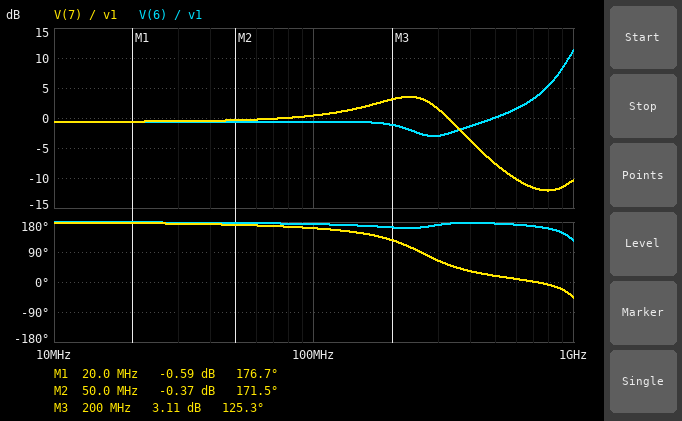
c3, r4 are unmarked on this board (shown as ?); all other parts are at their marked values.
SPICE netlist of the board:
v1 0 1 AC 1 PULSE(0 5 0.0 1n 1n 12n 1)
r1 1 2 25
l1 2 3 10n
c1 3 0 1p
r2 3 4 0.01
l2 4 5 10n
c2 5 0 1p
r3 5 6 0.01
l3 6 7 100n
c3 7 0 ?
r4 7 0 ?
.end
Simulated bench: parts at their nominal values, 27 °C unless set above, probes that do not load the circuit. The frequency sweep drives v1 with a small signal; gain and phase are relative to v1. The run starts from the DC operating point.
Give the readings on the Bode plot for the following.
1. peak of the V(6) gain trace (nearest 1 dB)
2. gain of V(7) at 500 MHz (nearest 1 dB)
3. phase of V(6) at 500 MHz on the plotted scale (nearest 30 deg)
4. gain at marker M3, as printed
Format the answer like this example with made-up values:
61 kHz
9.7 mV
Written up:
11 dB
-8 dB
180 deg
3.11 dB
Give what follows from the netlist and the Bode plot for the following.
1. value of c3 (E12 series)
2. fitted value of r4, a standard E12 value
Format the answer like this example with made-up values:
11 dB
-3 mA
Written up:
3.3 pF
330 Ω
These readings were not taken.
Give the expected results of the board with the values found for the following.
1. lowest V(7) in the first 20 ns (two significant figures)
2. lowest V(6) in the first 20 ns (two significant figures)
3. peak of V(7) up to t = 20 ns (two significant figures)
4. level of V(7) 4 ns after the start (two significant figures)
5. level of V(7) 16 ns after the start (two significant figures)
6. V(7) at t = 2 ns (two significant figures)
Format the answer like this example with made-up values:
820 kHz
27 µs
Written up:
-6.0 V
-5.0 V
1.4 V
-4.5 V
1.1 V
-5.3 V
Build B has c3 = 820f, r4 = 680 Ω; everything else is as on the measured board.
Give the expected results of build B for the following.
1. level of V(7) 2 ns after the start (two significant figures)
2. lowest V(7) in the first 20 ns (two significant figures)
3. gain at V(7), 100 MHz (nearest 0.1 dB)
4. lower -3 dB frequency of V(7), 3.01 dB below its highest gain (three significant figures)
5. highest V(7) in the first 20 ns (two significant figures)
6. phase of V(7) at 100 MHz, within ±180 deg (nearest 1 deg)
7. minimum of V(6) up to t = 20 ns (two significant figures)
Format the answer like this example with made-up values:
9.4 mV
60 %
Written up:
-5.5 V
-6.3 V
0 dB
300 MHz
1.5 V
171 deg
-5.2 V
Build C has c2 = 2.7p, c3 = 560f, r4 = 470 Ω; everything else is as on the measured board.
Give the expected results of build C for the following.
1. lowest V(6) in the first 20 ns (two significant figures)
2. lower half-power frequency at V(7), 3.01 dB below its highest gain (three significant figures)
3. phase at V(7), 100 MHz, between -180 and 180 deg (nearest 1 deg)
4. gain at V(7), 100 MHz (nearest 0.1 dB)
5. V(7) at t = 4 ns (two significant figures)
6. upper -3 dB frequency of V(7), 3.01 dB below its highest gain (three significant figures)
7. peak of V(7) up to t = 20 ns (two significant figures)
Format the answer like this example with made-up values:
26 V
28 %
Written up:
-5.6 V
391 MHz
167 deg
-0.2 dB
-4.7 V
829 MHz
1.3 V
